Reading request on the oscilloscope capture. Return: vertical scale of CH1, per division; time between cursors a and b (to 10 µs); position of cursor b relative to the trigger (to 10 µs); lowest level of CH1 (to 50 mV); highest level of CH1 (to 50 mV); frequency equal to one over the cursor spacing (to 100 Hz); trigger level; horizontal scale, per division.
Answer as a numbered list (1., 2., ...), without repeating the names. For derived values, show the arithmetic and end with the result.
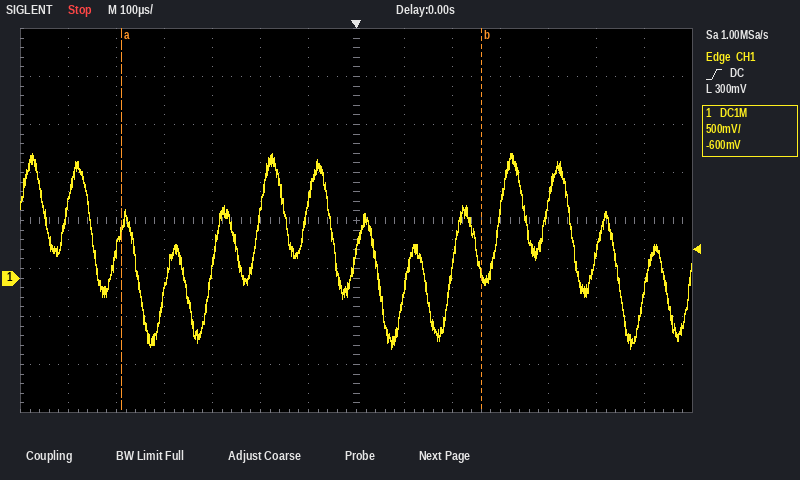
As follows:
1. 500 mV
2. 750 µs
3. +260 µs
4. -750 mV
5. 1.30 V
6. 1 / 750 µs ≈ 1.3 kHz
7. 300 mV
8. 100 µs
